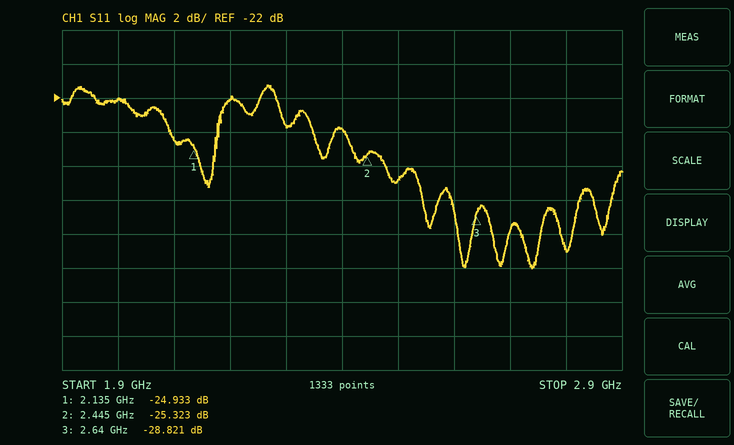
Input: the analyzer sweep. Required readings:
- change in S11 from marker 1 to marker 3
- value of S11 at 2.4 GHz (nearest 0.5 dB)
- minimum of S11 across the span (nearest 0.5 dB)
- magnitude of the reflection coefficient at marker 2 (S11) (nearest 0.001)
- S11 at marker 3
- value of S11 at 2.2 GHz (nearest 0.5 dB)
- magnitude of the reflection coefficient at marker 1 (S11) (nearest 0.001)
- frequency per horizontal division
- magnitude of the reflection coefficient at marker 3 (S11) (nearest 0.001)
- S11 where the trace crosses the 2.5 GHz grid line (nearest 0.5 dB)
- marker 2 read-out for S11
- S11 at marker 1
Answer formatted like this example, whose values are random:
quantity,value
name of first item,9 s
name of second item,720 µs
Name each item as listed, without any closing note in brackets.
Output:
quantity,value
change in S11 from marker 1 to marker 3,-3.888 dB
value of S11 at 2.4 GHz,-24.0 dB
minimum of S11 across the span,-32.0 dB
magnitude of the reflection coefficient at marker 2 (S11),0.054
S11 at marker 3,-28.821 dB
value of S11 at 2.2 GHz,-22.0 dB
magnitude of the reflection coefficient at marker 1 (S11),0.057
frequency per horizontal division,100 MHz
magnitude of the reflection coefficient at marker 3 (S11),0.036
S11 where the trace crosses the 2.5 GHz grid line,-27.0 dB
marker 2 read-out for S11,-25.323 dB
S11 at marker 1,-24.933 dB
